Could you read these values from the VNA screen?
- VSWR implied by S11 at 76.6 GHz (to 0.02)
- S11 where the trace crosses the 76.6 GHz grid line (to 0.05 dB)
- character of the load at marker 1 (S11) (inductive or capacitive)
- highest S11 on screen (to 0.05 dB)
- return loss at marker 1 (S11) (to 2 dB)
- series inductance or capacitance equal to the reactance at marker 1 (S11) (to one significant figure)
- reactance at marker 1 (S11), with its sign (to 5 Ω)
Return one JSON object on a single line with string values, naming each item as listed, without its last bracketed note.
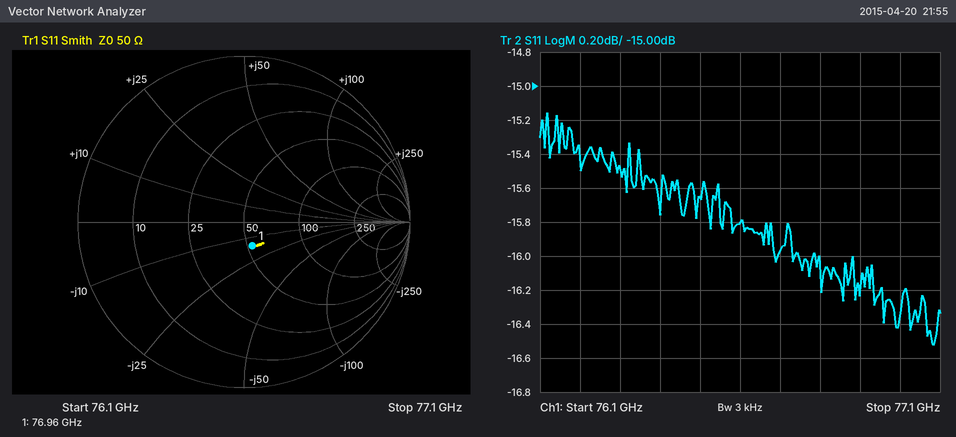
{"VSWR implied by S11 at 76.6 GHz": "1.38", "S11 where the trace crosses the 76.6 GHz grid line": "-15.80 dB", "character of the load at marker 1 (S11)": "capacitive", "highest S11 on screen": "-15.15 dB", "return loss at marker 1 (S11)": "16 dB", "series inductance or capacitance equal to the reactance at marker 1 (S11)": "100 fF", "reactance at marker 1 (S11), with its sign": "-15 Ω"}
